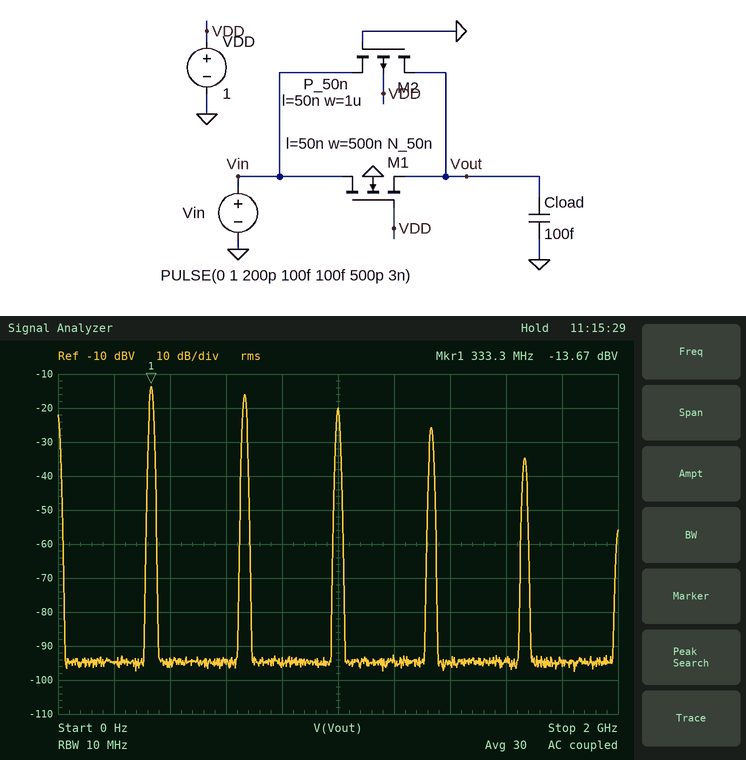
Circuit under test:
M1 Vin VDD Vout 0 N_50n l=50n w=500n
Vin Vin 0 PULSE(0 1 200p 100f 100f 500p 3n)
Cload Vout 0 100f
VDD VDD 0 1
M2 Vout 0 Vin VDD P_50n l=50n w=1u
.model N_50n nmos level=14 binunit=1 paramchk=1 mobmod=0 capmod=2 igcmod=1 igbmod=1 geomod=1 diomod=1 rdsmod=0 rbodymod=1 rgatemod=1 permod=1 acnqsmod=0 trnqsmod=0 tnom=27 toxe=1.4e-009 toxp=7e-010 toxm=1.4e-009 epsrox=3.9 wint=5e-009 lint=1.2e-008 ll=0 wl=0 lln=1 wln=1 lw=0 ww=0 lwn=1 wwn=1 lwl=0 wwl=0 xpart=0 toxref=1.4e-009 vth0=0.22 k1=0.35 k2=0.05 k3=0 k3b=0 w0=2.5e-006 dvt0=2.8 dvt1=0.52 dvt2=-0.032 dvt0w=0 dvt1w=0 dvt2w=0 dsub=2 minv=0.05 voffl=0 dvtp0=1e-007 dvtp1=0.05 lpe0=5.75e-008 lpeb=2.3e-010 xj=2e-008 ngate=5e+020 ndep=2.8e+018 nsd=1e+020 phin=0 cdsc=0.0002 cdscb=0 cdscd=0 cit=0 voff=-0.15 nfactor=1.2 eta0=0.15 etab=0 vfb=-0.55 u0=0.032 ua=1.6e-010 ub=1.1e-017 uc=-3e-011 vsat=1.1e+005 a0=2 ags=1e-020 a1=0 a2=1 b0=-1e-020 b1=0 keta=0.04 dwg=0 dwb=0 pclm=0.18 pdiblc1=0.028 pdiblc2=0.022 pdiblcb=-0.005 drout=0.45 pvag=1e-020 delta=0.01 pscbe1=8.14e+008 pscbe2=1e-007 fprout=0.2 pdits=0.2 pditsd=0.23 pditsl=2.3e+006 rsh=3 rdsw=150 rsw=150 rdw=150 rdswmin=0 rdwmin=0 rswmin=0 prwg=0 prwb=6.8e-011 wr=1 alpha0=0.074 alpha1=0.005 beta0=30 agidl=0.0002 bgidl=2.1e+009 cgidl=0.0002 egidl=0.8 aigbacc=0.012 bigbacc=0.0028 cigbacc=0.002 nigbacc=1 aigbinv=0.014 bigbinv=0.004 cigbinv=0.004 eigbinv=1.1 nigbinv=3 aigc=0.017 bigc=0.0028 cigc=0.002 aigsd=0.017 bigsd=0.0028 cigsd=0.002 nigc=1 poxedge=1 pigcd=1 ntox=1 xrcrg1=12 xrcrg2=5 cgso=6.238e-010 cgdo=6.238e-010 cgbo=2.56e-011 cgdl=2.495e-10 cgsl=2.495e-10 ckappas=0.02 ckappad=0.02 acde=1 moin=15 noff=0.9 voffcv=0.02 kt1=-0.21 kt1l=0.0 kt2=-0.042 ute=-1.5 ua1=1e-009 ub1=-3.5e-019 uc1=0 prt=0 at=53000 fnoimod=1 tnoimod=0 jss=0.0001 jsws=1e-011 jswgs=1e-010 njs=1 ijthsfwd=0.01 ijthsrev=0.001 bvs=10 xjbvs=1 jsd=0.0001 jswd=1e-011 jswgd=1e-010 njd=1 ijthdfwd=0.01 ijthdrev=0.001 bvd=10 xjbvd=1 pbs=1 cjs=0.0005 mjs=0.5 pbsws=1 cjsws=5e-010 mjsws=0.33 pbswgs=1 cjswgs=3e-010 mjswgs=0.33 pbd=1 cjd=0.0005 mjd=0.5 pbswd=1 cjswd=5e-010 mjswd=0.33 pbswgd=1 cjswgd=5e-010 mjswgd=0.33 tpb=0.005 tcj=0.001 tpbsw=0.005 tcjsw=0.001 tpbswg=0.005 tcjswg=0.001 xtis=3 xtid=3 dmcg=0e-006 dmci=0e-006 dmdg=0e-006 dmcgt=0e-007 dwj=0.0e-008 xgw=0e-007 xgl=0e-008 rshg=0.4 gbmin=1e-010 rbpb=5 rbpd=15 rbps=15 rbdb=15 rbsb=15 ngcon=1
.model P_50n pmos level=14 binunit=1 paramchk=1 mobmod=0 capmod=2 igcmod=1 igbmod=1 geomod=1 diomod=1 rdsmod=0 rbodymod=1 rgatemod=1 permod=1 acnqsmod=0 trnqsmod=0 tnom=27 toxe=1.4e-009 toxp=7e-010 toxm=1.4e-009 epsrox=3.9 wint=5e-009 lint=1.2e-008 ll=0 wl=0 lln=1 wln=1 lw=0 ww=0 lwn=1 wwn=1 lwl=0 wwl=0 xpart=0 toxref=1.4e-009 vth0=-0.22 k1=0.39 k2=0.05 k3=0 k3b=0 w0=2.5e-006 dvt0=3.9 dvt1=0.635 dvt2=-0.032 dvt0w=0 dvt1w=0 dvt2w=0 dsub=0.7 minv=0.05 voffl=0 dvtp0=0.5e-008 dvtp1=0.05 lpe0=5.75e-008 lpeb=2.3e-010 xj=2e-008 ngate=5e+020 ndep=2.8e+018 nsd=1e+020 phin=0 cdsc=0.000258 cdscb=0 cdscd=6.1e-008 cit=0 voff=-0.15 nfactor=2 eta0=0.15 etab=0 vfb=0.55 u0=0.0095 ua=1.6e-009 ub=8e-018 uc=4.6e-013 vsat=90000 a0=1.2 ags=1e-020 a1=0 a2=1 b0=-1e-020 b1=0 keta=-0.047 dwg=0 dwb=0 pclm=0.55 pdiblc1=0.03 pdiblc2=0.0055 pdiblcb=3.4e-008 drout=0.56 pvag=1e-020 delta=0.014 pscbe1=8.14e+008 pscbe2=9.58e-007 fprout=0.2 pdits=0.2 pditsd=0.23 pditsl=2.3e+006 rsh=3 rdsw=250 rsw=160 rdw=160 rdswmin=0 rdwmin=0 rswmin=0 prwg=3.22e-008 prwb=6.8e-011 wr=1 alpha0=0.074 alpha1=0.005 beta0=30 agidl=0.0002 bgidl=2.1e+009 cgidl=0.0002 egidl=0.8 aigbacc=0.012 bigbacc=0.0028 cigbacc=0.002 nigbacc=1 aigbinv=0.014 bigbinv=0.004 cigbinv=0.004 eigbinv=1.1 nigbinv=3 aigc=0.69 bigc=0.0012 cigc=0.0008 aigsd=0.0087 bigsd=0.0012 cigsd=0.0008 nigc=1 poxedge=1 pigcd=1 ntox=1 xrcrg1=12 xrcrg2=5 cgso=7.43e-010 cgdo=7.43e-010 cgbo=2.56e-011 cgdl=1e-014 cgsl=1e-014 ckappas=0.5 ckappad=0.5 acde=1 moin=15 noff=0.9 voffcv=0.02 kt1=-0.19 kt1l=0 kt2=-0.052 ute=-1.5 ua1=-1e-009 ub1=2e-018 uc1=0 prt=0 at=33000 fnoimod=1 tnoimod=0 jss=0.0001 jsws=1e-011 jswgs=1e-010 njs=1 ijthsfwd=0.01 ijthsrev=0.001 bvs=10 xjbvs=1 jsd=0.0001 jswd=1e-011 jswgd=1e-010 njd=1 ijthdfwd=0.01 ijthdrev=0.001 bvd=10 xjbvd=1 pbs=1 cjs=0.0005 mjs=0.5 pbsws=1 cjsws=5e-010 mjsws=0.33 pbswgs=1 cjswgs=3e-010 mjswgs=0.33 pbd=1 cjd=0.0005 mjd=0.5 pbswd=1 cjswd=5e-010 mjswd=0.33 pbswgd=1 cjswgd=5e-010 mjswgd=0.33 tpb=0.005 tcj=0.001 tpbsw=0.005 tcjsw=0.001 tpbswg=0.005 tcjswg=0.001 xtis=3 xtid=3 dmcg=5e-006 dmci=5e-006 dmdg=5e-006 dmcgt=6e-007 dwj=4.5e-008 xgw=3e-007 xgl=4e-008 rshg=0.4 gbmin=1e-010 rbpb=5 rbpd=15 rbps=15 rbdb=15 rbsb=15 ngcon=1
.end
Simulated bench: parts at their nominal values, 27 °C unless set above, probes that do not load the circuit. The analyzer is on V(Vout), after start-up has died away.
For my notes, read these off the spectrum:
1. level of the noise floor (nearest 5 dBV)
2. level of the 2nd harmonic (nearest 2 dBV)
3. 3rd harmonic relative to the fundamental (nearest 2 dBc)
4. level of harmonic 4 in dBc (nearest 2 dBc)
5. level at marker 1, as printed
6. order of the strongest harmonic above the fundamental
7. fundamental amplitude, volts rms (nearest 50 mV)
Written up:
-95 dBV
-16 dBV
-6 dBc
-12 dBc
-13.67 dBV
2
200 mV
